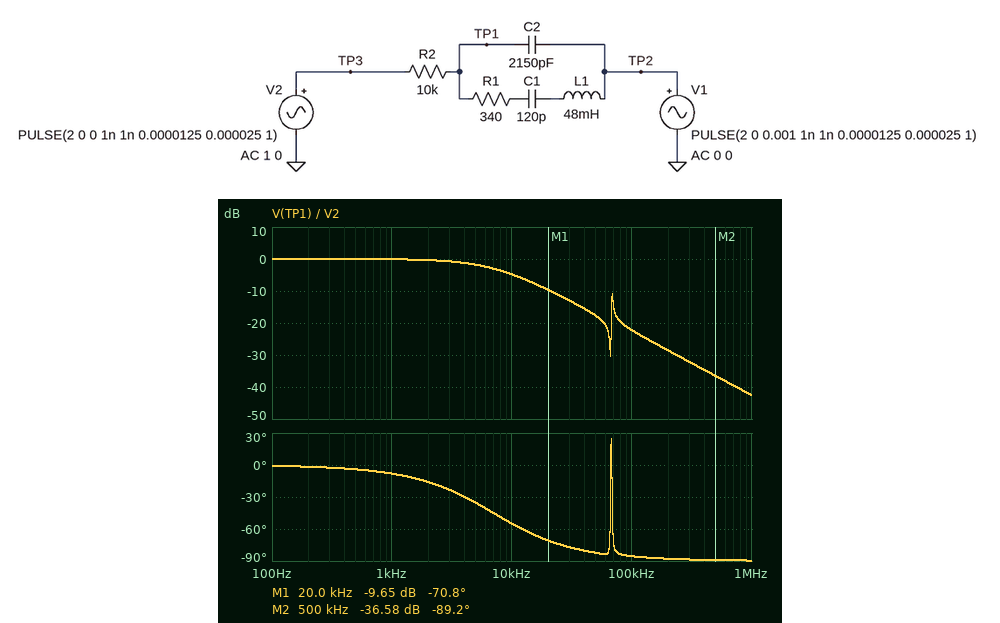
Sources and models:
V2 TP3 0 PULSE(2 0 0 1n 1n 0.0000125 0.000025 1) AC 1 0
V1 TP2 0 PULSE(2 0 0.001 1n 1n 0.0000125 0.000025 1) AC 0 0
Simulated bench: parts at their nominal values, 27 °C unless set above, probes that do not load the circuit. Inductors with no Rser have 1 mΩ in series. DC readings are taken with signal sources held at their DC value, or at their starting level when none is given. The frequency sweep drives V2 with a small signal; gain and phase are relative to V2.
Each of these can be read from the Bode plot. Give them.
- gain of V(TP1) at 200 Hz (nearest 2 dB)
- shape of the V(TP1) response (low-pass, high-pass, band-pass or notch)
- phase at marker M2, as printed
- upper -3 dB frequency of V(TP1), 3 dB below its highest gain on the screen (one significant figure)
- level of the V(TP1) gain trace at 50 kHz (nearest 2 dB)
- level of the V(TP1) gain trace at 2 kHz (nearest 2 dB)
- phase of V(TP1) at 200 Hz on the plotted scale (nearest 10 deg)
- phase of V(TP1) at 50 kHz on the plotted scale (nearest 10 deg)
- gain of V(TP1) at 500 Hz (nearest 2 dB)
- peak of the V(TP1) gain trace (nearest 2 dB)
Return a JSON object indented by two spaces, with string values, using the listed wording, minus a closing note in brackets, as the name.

{
  "gain of V(TP1) at 200 Hz": "0 dB",
  "shape of the V(TP1) response": "low-pass",
  "phase at marker M2, as printed": "-89.2 deg",
  "upper -3 dB frequency of V(TP1), 3 dB below its highest gain on the screen": "7 kHz",
  "level of the V(TP1) gain trace at 50 kHz": "-18 dB",
  "level of the V(TP1) gain trace at 2 kHz": "0 dB",
  "phase of V(TP1) at 200 Hz on the plotted scale": "0 deg",
  "phase of V(TP1) at 50 kHz on the plotted scale": "-80 deg",
  "gain of V(TP1) at 500 Hz": "0 dB",
  "peak of the V(TP1) gain trace": "0 dB"
}
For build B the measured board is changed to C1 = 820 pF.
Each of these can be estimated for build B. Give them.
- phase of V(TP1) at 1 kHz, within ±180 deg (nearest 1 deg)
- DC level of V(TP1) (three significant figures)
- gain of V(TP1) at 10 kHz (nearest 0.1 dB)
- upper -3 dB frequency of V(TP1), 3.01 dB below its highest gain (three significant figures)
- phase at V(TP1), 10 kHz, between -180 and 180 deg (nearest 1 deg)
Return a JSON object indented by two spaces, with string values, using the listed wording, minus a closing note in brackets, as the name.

{
  "phase of V(TP1) at 1 kHz, within ±180 deg": "-11 deg",
  "DC level of V(TP1)": "2.00 V",
  "gain of V(TP1) at 10 kHz": "-6.9 dB",
  "upper -3 dB frequency of V(TP1), 3.01 dB below its highest gain": "5.28 kHz",
  "phase at V(TP1), 10 kHz, between -180 and 180 deg": "-63 deg"
}
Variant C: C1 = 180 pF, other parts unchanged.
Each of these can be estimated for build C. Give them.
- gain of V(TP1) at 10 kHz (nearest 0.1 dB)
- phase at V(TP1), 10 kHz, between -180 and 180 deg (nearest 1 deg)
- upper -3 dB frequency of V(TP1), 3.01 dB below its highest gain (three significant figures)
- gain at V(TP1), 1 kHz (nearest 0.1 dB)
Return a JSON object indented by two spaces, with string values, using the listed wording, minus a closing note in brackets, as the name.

{
  "gain of V(TP1) at 10 kHz": "-5.0 dB",
  "phase at V(TP1), 10 kHz, between -180 and 180 deg": "-56 deg",
  "upper -3 dB frequency of V(TP1), 3.01 dB below its highest gain": "6.82 kHz",
  "gain at V(TP1), 1 kHz": "-0.1 dB"
}
